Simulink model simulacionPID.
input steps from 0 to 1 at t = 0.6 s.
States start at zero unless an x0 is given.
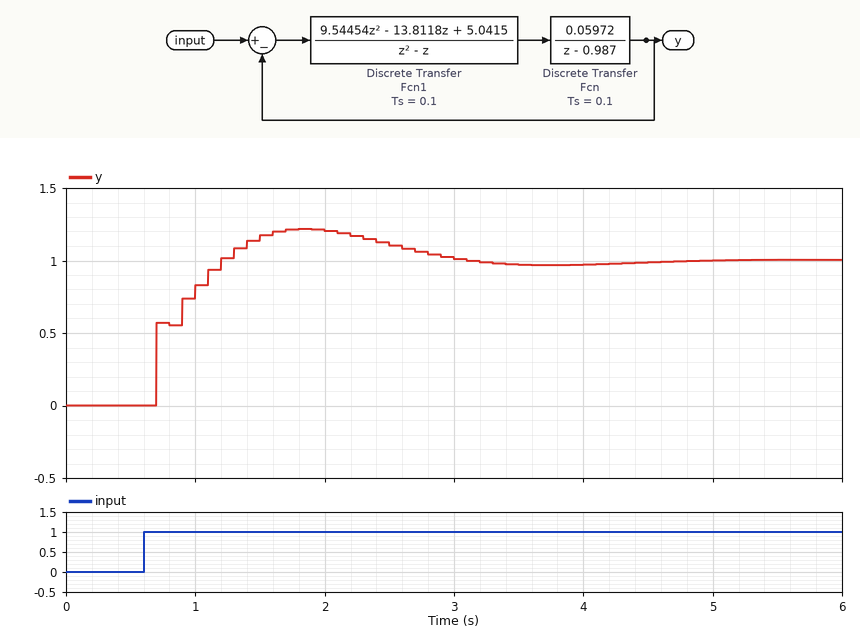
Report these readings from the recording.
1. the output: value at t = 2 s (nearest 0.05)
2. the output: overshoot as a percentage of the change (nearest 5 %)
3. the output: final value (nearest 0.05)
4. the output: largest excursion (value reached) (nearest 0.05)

1.20
20 %
1.00
1.20
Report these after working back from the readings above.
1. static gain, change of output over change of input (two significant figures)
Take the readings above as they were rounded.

1.0
